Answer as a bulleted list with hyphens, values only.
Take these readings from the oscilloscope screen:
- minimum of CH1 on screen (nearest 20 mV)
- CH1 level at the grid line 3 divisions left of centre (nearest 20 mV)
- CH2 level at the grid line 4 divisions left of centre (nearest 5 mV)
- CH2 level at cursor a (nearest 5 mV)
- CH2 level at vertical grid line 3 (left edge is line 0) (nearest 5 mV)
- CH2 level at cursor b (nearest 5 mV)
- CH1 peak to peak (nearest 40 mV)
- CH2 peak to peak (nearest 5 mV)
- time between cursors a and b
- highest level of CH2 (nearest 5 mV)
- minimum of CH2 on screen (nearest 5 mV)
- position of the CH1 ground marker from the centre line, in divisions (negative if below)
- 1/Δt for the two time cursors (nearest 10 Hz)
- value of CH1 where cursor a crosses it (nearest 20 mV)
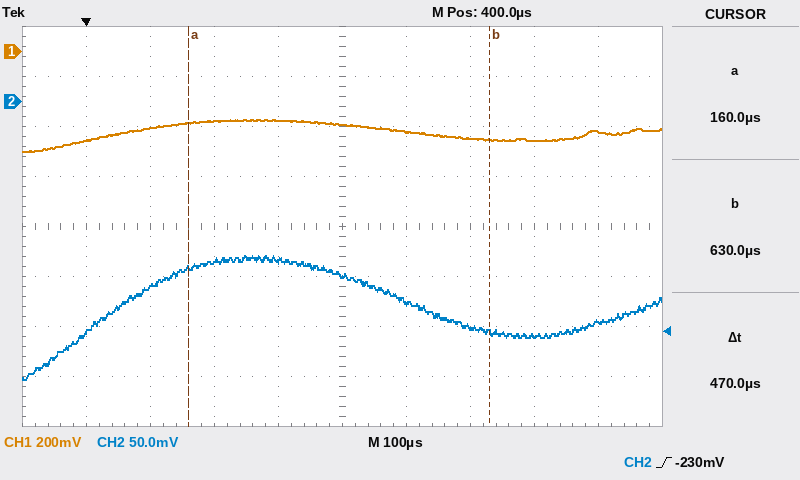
- -400 mV
- -300 mV
- -230 mV
- -165 mV
- -160 mV
- -230 mV
- 120 mV
- 125 mV
- 470 µs
- -155 mV
- -280 mV
- +3.5 div
- 2.13 kHz
- -280 mV
